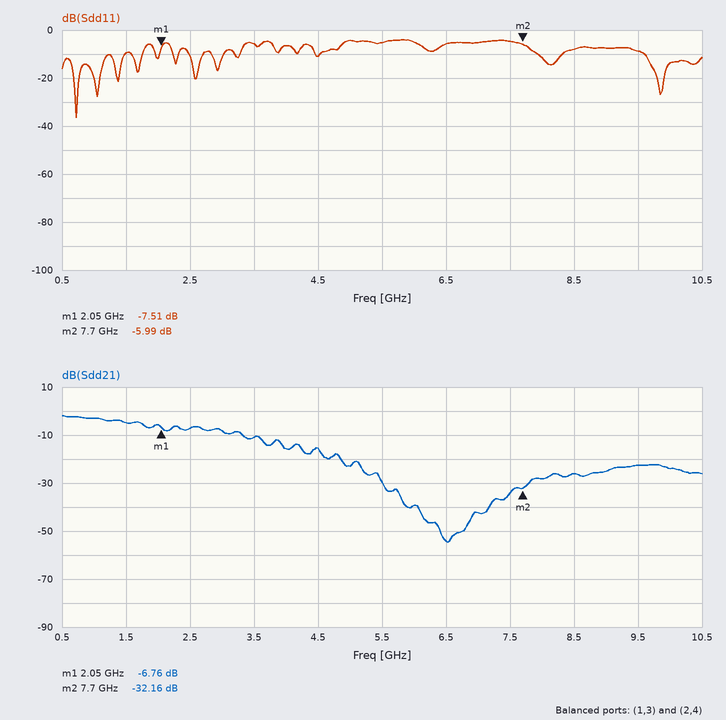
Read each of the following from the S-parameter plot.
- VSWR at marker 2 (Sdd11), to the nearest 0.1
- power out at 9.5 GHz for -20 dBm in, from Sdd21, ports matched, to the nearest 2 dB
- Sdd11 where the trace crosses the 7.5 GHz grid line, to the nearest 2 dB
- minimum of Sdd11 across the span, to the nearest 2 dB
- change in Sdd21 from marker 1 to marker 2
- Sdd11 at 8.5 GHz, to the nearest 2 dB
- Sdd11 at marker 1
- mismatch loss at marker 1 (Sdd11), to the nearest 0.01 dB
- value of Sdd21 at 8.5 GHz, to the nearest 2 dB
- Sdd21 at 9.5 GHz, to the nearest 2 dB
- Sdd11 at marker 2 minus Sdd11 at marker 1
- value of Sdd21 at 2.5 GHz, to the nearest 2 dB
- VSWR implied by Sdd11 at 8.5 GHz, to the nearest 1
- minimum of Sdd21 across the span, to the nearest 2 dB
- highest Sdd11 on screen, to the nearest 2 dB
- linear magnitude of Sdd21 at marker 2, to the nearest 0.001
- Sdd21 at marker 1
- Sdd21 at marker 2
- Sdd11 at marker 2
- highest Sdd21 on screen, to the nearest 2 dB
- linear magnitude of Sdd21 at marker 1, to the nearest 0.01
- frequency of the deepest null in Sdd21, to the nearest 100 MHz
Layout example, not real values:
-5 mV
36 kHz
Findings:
3.0
-42 dBm
-4 dB
-36 dB
-25.40 dB
-8 dB
-7.51 dB
0.85 dB
-26 dB
-22 dB
1.52 dB
-8 dB
2
-54 dB
-4 dB
0.025
-6.76 dB
-32.16 dB
-5.99 dB
-2 dB
0.46
6.5 GHz
